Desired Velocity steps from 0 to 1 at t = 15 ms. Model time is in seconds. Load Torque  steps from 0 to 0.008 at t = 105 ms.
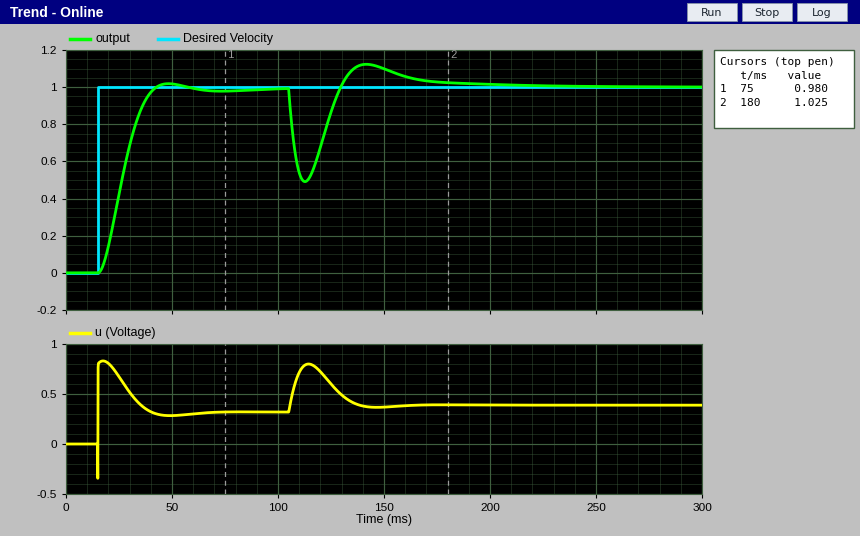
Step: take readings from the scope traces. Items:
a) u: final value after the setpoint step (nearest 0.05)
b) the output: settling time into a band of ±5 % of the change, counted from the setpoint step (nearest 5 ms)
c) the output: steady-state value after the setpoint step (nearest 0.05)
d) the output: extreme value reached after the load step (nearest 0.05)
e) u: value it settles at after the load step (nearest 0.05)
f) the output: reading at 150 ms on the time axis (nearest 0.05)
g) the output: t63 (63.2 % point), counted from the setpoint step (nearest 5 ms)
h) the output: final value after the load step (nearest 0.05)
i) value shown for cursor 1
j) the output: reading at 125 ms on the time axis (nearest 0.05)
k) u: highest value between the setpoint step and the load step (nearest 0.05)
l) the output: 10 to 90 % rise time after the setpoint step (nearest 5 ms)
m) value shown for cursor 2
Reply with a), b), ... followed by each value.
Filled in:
a) 0.30
b) 25 ms
c) 1.00
d) 0.50
e) 0.40
f) 1.10
g) 15 ms
h) 1.00
i) 0.980
j) 0.85
k) 0.85
l) 15 ms
m) 1.025
